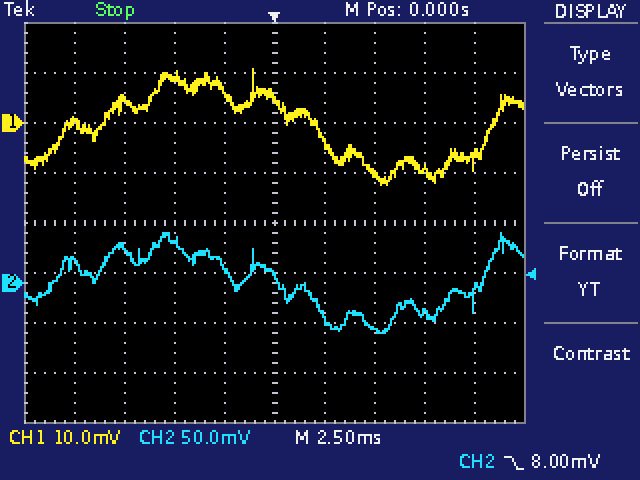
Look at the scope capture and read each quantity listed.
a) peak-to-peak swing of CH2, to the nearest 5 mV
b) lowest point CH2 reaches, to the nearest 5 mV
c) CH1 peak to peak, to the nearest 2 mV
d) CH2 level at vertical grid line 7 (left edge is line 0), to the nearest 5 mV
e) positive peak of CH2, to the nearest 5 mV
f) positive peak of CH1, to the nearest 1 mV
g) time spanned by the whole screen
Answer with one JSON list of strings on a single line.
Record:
["100 mV", "-50 mV", "24 mV", "-45 mV", "50 mV", "11 mV", "25 ms"]
